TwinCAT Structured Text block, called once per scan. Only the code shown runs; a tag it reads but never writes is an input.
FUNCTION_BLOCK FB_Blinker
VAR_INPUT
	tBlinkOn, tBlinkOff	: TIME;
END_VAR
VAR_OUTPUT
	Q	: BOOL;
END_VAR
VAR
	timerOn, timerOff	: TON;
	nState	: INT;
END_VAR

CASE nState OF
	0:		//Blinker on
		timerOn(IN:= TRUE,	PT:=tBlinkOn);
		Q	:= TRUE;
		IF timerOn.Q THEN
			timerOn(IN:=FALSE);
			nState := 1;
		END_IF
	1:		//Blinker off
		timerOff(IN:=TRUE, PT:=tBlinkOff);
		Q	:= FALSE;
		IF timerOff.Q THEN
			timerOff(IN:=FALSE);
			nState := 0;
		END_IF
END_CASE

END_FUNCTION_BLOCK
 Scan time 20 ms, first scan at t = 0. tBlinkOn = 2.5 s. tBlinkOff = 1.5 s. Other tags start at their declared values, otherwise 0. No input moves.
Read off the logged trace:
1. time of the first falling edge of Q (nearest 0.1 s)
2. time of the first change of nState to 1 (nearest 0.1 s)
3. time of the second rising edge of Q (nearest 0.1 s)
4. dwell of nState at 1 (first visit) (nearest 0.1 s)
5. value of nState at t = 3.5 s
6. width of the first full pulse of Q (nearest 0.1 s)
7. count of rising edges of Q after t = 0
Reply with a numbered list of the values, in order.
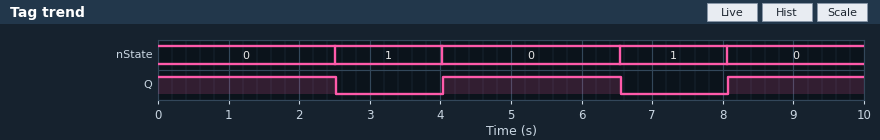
1. 2.5 s
2. 2.5 s
3. 8.1 s
4. 1.5 s
5. 1
6. 2.5 s
7. 2
